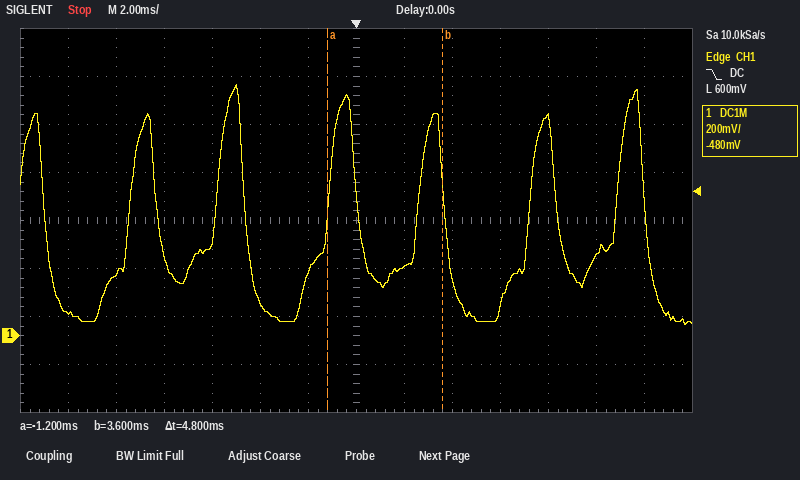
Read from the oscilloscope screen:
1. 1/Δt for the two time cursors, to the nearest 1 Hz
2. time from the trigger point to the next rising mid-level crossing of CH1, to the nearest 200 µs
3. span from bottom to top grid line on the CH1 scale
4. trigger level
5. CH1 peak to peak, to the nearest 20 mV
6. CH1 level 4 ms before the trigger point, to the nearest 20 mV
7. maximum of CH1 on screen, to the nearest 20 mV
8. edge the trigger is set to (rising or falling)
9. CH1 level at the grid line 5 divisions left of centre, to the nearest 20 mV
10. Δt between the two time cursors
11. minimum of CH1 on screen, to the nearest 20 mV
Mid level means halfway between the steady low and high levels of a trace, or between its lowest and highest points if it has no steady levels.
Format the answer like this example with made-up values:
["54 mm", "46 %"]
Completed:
["208 Hz", "2.6 ms", "1.6 V", "600 mV", "1.00 V", "140 mV", "1.04 V", "falling", "260 mV", "4.8 ms", "40 mV"]
